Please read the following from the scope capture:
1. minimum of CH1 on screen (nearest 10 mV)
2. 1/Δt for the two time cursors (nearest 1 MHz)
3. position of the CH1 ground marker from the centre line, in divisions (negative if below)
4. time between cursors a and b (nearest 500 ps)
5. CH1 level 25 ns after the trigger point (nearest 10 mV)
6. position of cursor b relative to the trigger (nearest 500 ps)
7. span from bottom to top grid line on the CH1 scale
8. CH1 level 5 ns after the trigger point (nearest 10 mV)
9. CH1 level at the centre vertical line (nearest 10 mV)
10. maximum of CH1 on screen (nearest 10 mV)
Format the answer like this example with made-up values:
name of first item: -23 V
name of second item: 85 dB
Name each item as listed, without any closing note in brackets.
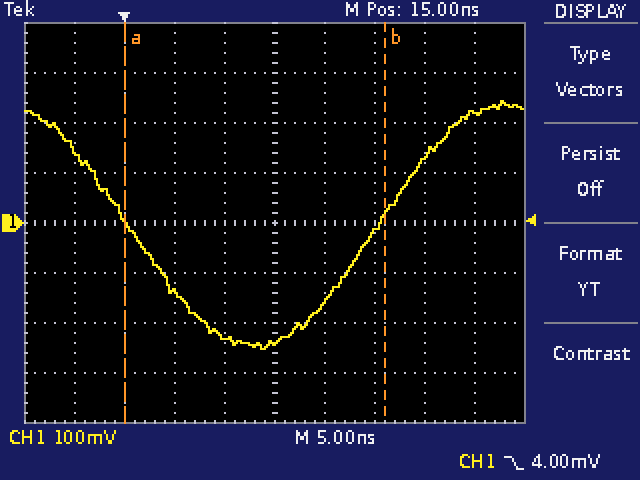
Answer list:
minimum of CH1 on screen: -250 mV
1/Δt for the two time cursors: 38 MHz
position of the CH1 ground marker from the centre line, in divisions: 0.0 div
time between cursors a and b: 26.0 ns
CH1 level 25 ns after the trigger point: -20 mV
position of cursor b relative to the trigger: +26.0 ns
span from bottom to top grid line on the CH1 scale: 800 mV
CH1 level 5 ns after the trigger point: -140 mV
CH1 level at the centre vertical line: -240 mV
maximum of CH1 on screen: 240 mV
